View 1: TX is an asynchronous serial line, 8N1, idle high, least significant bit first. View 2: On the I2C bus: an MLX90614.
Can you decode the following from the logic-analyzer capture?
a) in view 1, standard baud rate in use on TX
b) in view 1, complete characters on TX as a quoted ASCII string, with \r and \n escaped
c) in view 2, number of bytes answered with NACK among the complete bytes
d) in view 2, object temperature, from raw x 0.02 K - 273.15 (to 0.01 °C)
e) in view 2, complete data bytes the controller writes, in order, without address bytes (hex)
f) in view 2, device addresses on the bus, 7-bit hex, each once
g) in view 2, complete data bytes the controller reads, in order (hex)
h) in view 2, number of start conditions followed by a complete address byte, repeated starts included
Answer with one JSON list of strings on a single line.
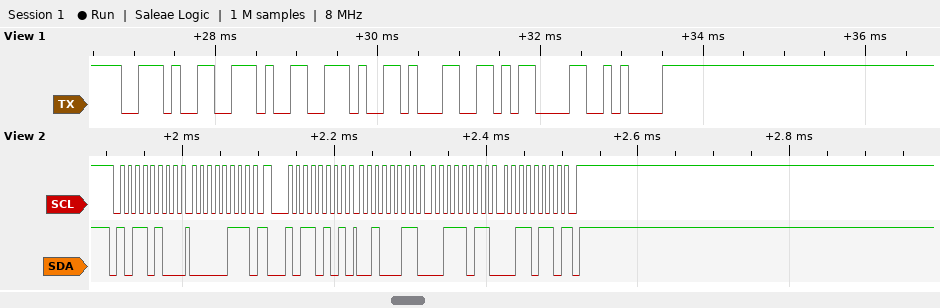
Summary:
["9600 baud", "\"...1\\r\\n\"", "1", "29.63 °C", "07", "0x5A", "23 3B 36", "2"]
